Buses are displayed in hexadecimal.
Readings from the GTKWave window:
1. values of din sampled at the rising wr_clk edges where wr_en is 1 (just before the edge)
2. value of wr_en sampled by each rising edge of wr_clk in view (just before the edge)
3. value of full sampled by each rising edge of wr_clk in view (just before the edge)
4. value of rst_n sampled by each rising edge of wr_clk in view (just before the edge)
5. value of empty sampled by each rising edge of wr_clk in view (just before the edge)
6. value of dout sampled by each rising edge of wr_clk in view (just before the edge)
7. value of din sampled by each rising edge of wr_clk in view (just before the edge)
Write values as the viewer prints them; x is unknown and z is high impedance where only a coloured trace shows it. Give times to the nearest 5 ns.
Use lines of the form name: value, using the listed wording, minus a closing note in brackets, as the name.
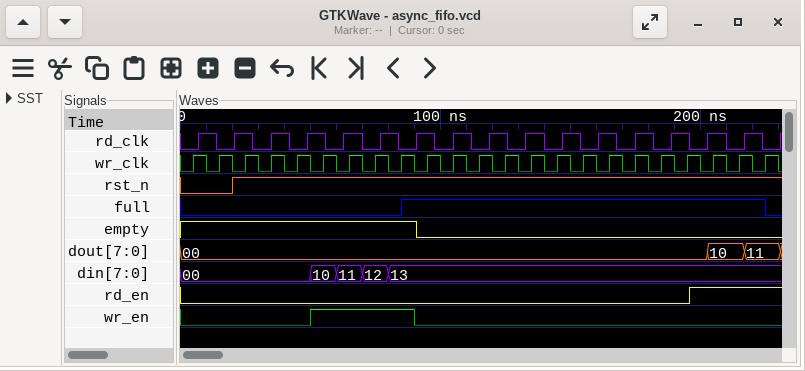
values of din sampled at the rising wr_clk edges where wr_en is 1: 10, 11, 12, 13
value of wr_en sampled by each rising edge of wr_clk in view: 0 0 0 0 0 1 1 1 1 0 0 0 0 0 0 0 0 0 0 0 0 0 0
value of full sampled by each rising edge of wr_clk in view: 0 0 0 0 0 0 0 0 0 1 1 1 1 1 1 1 1 1 1 1 1 1 1
value of rst_n sampled by each rising edge of wr_clk in view: 0 0 1 1 1 1 1 1 1 1 1 1 1 1 1 1 1 1 1 1 1 1 1
value of empty sampled by each rising edge of wr_clk in view: 1 1 1 1 1 1 1 1 1 0 0 0 0 0 0 0 0 0 0 0 0 0 0
value of dout sampled by each rising edge of wr_clk in view: 00, 00, 00, 00, 00, 00, 00, 00, 00, 00, 00, 00, 00, 00, 00, 00, 00, 00, 00, 00, 10, 10, 11
value of din sampled by each rising edge of wr_clk in view: 00, 00, 00, 00, 00, 10, 11, 12, 13, 13, 13, 13, 13, 13, 13, 13, 13, 13, 13, 13, 13, 13, 13
